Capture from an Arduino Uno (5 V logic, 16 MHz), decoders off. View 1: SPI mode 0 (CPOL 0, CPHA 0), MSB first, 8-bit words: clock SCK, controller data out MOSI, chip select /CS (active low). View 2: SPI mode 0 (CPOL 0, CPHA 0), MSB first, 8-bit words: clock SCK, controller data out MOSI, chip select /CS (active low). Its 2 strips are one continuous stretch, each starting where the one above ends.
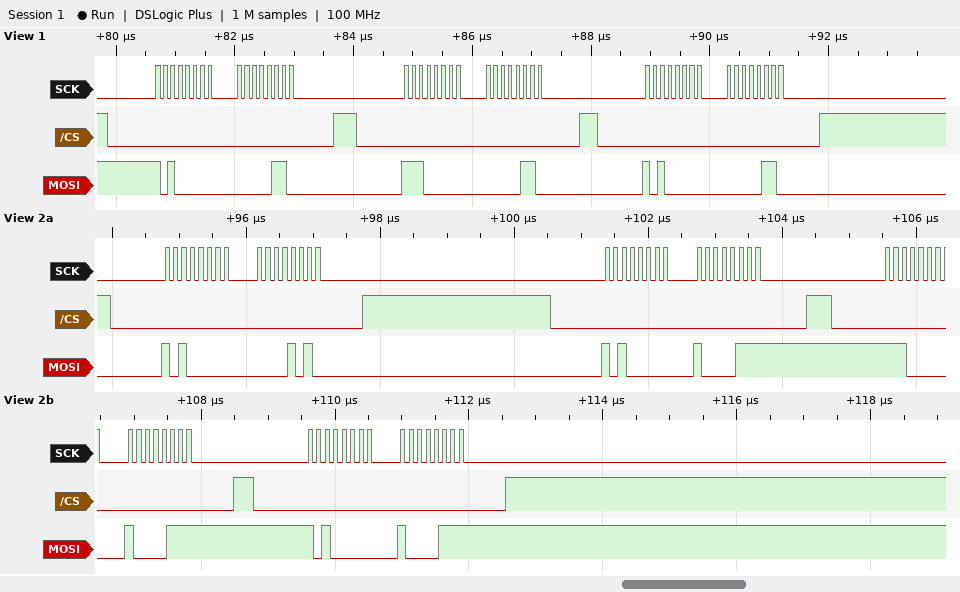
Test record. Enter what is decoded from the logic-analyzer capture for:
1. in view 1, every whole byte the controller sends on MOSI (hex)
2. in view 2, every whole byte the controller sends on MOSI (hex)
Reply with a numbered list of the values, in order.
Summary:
1. A0 06 E0 06 A0 06
2. 0xA0 0x0A 0xA0 0x87 0xE0 0x87 0xA0 0x87
